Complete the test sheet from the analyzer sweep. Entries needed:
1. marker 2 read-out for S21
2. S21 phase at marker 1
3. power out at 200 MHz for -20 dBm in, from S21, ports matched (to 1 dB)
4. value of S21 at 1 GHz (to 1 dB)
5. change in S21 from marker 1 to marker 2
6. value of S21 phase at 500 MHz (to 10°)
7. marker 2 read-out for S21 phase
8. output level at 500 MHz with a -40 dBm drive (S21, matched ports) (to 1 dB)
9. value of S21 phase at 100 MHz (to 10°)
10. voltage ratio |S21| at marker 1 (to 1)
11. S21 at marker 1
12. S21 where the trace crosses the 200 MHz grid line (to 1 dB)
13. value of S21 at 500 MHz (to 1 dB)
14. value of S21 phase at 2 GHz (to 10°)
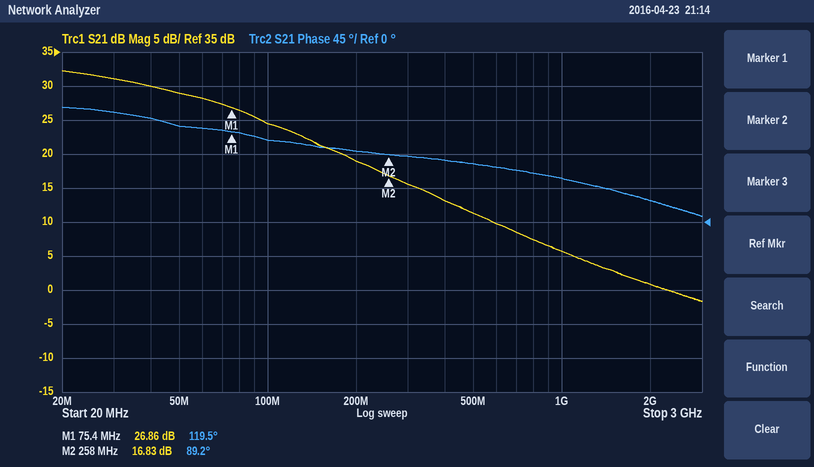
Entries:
16.83 dB
119.5°
-1 dBm
6 dB
-10.03 dB
80°
89.2°
-29 dBm
110°
22
26.86 dB
19 dB
11 dB
30°
